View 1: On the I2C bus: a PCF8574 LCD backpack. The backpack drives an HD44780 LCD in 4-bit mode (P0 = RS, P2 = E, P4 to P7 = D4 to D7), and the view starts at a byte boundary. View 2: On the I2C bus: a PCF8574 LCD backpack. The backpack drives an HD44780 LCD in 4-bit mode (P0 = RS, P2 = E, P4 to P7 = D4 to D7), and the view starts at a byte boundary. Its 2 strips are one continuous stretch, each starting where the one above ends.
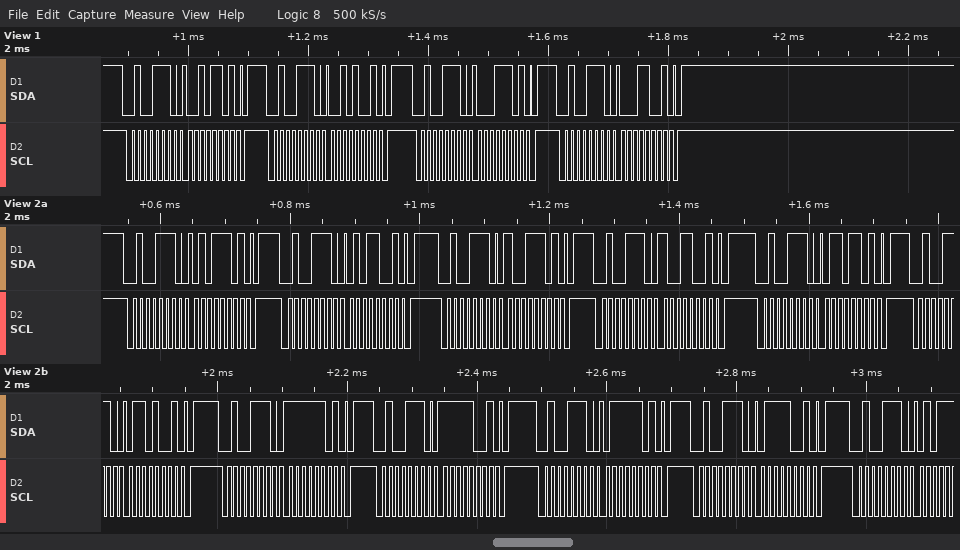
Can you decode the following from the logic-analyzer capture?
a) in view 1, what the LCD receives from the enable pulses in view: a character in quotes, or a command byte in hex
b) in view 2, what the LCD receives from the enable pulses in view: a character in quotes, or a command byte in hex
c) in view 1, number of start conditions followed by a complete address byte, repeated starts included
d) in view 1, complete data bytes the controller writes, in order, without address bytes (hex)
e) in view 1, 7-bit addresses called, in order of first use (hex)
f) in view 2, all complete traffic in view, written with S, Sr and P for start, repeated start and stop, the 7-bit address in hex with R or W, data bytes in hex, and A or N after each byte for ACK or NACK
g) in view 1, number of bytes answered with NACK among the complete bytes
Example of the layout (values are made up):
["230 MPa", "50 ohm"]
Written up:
["'!'", "'Y' 'o'", "4", "2D 29 1D 19", "0x27", "S 27W A 5D A P S 27W A 59 A P S 27W A 9D A P S 27W A 99 A P S 27W A 6D A P S 27W A 69 A P S 27W A FD A P S 27W A F9 A P S 27W A 7D A P S 27W A 79 A P S 27W A", "0"]
